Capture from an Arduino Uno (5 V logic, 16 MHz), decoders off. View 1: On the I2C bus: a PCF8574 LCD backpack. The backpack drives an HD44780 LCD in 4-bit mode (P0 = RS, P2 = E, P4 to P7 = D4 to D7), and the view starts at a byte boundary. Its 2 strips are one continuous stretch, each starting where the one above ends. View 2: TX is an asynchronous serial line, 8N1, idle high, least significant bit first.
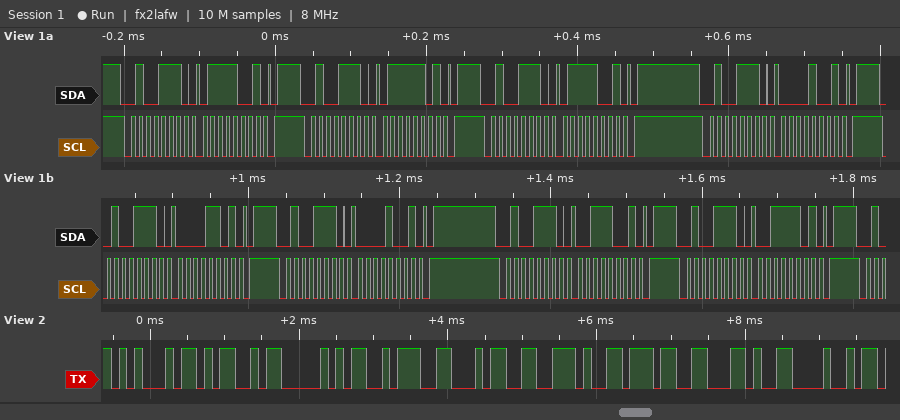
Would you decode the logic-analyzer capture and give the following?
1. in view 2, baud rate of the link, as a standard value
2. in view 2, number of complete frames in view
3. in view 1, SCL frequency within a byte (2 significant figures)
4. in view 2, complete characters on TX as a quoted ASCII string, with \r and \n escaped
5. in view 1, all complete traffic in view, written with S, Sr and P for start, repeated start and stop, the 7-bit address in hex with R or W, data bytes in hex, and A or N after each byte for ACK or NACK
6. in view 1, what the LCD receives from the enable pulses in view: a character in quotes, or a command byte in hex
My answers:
9600 baud
9
100 kHz
"EMP:4.7,H"
S 27W A 79 A P S 27W A 7D A P S 27W A 79 A P S 27W A 09 A P S 27W A 0D A P S 27W A 09 A P S 27W A 39 A P S 27W A 3D A P
'p'
